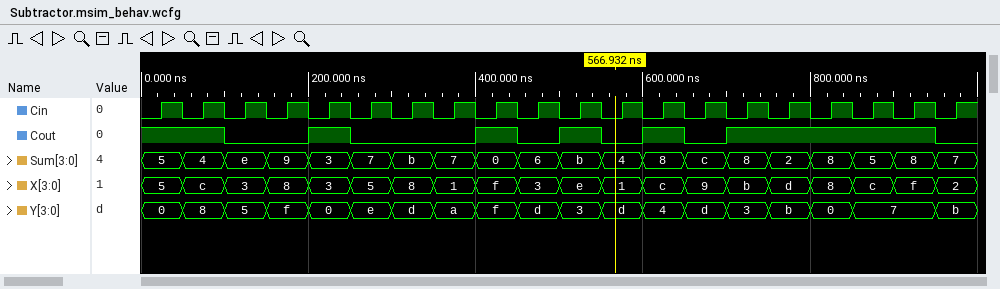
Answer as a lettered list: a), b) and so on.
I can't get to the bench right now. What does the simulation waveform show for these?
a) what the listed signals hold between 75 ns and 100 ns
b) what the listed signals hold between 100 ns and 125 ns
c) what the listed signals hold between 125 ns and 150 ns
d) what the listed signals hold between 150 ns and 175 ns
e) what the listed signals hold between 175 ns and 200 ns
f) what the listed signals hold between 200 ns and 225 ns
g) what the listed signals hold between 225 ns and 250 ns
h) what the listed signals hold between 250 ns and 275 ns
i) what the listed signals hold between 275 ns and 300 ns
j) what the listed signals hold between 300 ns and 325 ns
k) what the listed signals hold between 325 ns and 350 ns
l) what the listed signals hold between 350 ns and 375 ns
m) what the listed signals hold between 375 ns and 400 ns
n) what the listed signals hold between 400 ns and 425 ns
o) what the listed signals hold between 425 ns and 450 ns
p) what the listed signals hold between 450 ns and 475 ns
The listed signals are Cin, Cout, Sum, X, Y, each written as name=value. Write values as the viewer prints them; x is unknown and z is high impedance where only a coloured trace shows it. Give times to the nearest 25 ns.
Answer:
a) Cin=1, Cout=1, Sum=4, X=c, Y=8
b) Cin=0, Cout=0, Sum=e, X=3, Y=5
c) Cin=1, Cout=0, Sum=e, X=3, Y=5
d) Cin=0, Cout=0, Sum=9, X=8, Y=f
e) Cin=1, Cout=0, Sum=9, X=8, Y=f
f) Cin=0, Cout=1, Sum=3, X=3, Y=0
g) Cin=1, Cout=1, Sum=3, X=3, Y=0
h) Cin=0, Cout=0, Sum=7, X=5, Y=e
i) Cin=1, Cout=0, Sum=7, X=5, Y=e
j) Cin=0, Cout=0, Sum=b, X=8, Y=d
k) Cin=1, Cout=0, Sum=b, X=8, Y=d
l) Cin=0, Cout=0, Sum=7, X=1, Y=a
m) Cin=1, Cout=0, Sum=7, X=1, Y=a
n) Cin=0, Cout=1, Sum=0, X=f, Y=f
o) Cin=1, Cout=1, Sum=0, X=f, Y=f
p) Cin=0, Cout=0, Sum=6, X=3, Y=d
